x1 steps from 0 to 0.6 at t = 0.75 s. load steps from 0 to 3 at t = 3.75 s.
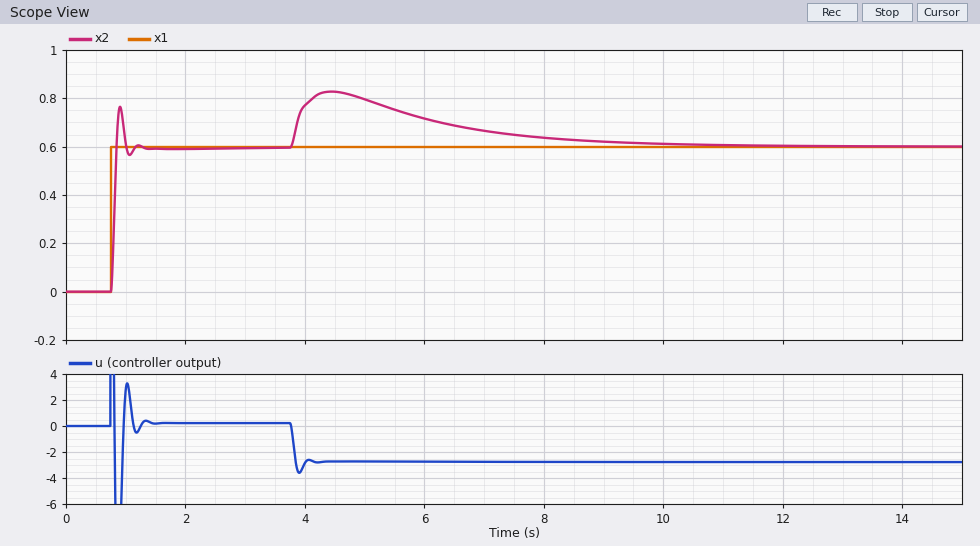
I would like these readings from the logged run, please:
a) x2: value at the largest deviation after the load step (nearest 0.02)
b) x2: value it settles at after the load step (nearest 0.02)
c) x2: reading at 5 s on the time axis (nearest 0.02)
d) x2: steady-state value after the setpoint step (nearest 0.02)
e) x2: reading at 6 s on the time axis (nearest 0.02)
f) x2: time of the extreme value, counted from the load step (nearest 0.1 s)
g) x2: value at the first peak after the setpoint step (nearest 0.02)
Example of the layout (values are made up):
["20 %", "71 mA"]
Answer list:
["0.82", "0.60", "0.80", "0.60", "0.72", "0.7 s", "0.76"]
